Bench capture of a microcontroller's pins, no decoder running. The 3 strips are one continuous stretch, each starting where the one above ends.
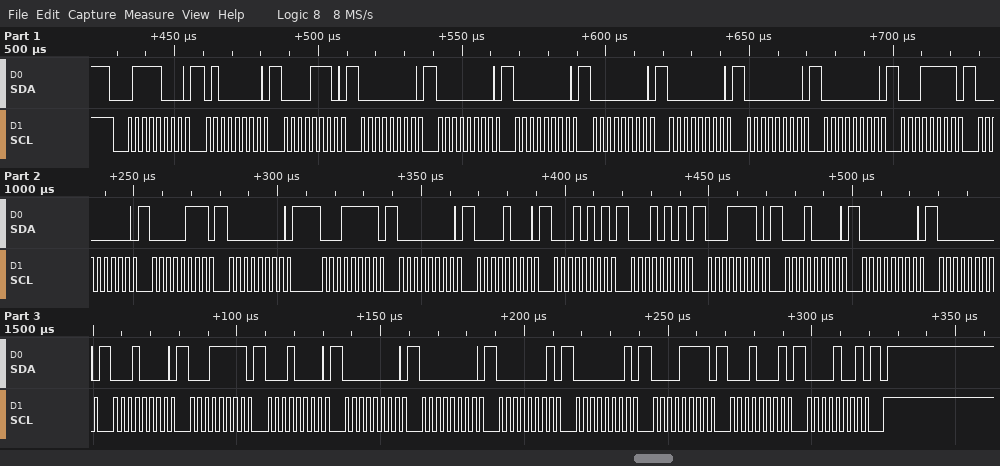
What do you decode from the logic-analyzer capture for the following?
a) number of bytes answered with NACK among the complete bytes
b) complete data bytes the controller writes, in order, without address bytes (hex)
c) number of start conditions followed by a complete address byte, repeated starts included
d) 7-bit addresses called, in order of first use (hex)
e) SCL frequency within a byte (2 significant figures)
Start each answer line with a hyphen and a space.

- 0
- 40 0E 00 00 00 00 00 00 00 1F 00 07 00 1F 00 08 15 15 1E 10 00 00 10 1F 10 00 00 01 01 0F 11 09
- 1
- 0x3C
- 400 kHz
